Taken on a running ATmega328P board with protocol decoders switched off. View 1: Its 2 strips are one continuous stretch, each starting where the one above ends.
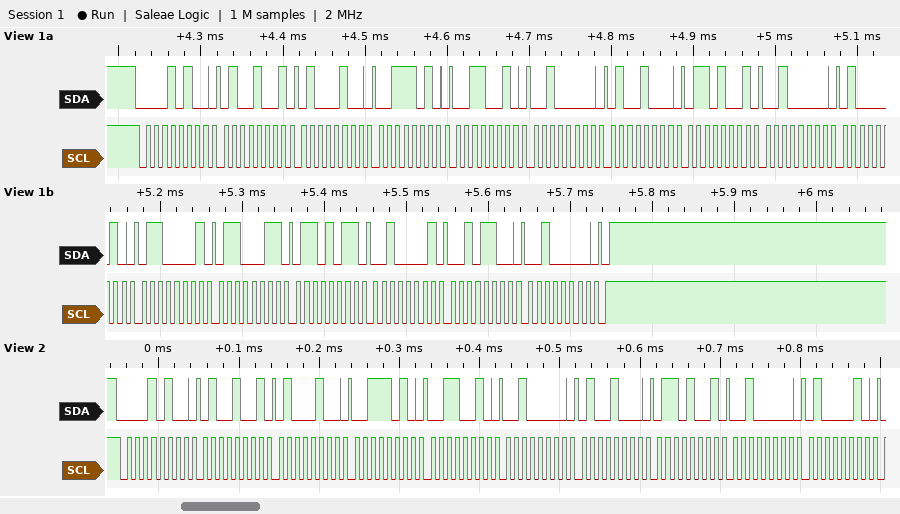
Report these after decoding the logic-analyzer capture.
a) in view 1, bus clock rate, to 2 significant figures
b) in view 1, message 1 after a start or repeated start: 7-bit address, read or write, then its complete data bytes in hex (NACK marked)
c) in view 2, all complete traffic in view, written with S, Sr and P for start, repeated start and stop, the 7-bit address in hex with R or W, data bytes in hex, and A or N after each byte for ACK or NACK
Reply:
100 kHz
0x0A write: 49 44 3A 32 20 48 69 20 42 61 63 6B 21 2C 20
S 0AW A 49 A 44 A 3A A 32 A 20 A 48 A 69 A 20 A 42 A
